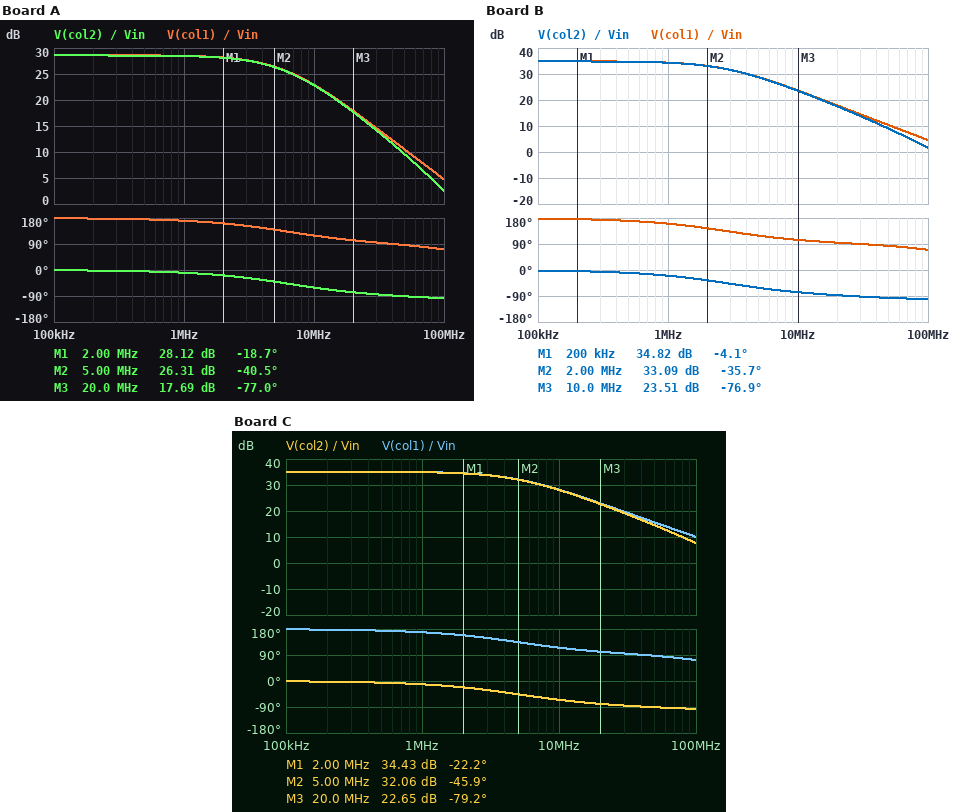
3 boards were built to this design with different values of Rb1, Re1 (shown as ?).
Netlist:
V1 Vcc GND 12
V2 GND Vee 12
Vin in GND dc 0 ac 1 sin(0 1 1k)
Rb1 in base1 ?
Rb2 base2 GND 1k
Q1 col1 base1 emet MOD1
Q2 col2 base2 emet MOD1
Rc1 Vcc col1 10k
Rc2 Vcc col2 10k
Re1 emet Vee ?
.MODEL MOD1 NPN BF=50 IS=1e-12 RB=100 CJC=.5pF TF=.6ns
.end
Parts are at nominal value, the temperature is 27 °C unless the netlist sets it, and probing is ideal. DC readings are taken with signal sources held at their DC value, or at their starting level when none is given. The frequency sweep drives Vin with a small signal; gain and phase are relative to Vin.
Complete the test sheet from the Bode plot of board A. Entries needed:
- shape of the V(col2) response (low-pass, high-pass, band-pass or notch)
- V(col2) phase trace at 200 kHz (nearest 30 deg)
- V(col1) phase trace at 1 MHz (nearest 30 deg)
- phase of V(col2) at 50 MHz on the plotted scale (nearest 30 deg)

low-pass
0 deg
180 deg
-90 deg
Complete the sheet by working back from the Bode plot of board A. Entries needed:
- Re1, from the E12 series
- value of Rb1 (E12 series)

33 kΩ
2.2 kΩ
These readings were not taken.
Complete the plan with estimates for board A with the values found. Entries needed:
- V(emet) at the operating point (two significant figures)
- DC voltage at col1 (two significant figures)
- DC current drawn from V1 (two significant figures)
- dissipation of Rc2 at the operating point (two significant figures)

-500 mV
10 V
340 µA
330 µW
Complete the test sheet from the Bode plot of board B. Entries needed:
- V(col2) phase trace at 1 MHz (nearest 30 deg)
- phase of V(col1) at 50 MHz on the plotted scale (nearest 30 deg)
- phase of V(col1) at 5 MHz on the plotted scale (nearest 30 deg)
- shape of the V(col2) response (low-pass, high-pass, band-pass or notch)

-30 deg
90 deg
120 deg
low-pass
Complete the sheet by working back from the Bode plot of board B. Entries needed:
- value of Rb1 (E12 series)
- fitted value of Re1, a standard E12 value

2.2 kΩ
12 kΩ
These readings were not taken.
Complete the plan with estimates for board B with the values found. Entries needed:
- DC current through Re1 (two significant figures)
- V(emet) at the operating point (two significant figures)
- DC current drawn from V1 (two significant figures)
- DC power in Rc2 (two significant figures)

960 µA
-530 mV
940 µA
2.8 mW
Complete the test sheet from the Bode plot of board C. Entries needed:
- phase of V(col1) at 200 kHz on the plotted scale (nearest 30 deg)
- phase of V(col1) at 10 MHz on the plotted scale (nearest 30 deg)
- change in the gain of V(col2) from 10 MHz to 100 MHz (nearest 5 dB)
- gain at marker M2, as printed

180 deg
120 deg
-20 dB
32.06 dB
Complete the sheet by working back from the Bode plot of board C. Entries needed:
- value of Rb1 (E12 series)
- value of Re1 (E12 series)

680 Ω
15 kΩ
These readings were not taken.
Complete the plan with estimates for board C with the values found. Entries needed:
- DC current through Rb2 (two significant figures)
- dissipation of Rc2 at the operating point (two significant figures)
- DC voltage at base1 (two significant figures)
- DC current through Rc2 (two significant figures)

7.2 µA
1.3 mW
-5.3 mV
360 µA
